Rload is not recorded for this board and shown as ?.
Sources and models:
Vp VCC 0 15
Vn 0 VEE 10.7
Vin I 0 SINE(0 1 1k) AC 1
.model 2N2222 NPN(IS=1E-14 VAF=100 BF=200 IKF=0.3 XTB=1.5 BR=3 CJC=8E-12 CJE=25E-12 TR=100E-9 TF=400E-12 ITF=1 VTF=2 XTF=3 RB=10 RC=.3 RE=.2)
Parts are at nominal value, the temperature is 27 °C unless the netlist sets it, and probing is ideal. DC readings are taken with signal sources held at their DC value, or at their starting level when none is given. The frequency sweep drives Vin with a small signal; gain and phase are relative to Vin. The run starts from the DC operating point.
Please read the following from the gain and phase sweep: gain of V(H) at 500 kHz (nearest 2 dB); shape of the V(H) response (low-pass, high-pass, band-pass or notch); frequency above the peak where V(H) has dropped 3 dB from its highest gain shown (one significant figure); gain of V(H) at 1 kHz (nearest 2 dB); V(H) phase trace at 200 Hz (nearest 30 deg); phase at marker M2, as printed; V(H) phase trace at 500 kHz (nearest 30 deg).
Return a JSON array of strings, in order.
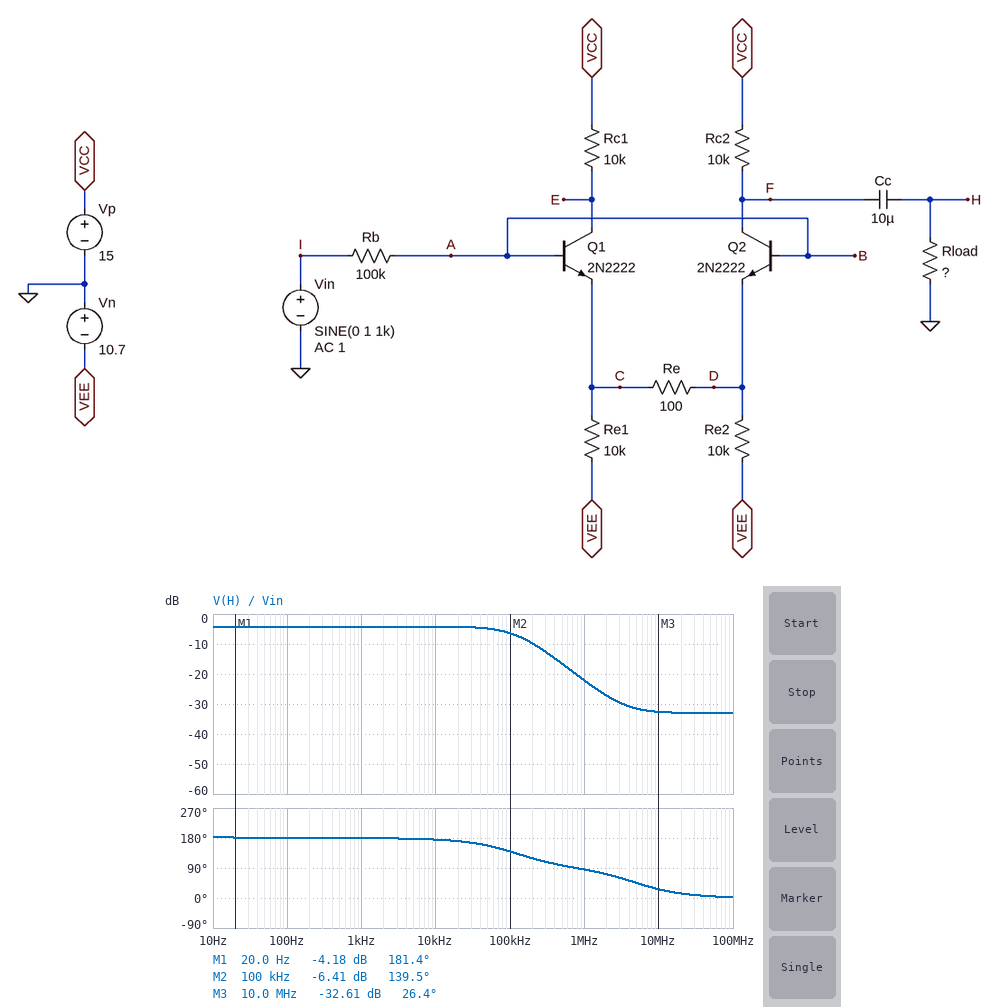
["-16 dB", "low-pass", "100 kHz", "-4 dB", "180 deg", "139.5 deg", "90 deg"]
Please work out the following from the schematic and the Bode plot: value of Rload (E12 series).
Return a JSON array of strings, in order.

["22 kΩ"]
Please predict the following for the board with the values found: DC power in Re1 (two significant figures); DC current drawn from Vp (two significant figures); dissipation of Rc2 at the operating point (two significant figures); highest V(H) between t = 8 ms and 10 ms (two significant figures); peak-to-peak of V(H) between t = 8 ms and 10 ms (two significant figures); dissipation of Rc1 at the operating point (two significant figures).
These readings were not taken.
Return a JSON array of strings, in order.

["8.4 mW", "1.8 mA", "8.4 mW", "620 mV", "1.2 V", "8.4 mW"]
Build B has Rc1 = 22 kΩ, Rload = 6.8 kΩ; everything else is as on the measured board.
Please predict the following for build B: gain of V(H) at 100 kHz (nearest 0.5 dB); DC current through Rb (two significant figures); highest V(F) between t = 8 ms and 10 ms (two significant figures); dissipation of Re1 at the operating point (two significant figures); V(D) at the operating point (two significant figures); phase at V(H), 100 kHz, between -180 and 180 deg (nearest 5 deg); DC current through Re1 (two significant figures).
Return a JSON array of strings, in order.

["-24.0 dB", "18 µA", "6.7 V", "6.8 mW", "-2.5 V", "170 deg", "820 µA"]
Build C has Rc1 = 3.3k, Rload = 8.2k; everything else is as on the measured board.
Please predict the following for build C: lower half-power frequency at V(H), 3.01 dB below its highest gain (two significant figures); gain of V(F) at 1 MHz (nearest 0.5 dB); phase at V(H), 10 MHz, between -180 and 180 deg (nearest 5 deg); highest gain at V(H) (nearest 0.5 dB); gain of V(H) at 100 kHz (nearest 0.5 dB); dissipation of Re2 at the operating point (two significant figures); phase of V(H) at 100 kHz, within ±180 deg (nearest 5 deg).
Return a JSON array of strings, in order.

["880 mHz", "-23.0 dB", "15 deg", "-8.0 dB", "-9.0 dB", "8.5 mW", "150 deg"]
